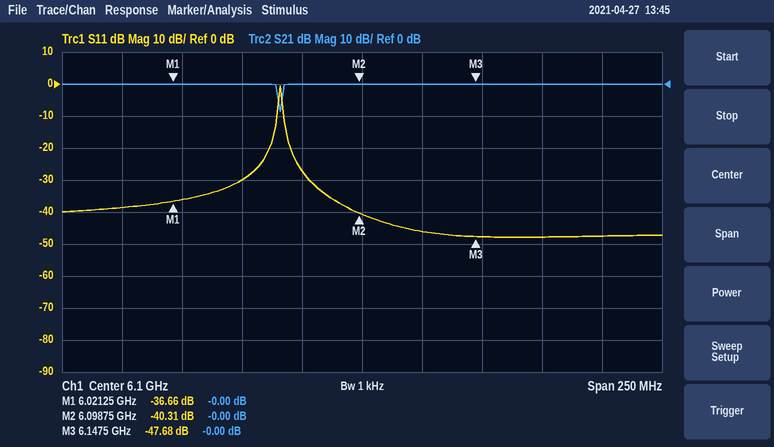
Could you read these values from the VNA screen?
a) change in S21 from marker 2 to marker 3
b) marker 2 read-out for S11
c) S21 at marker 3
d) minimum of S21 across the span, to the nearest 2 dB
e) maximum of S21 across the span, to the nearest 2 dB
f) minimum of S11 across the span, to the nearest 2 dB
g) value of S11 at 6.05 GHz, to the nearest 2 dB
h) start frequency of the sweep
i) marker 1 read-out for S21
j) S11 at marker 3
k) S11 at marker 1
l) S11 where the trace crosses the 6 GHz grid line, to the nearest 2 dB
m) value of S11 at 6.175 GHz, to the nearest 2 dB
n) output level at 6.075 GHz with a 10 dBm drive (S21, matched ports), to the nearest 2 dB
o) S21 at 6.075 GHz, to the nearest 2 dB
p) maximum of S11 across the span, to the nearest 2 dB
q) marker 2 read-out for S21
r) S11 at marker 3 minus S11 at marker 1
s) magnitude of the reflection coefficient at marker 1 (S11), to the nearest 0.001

0.00 dB
-40.31 dB
-0.00 dB
-8 dB
0 dB
-48 dB
-30 dB
5.975 GHz
-0.00 dB
-47.68 dB
-36.66 dB
-38 dB
-48 dB
10 dBm
0 dB
0 dB
-0.00 dB
-11.02 dB
0.015
